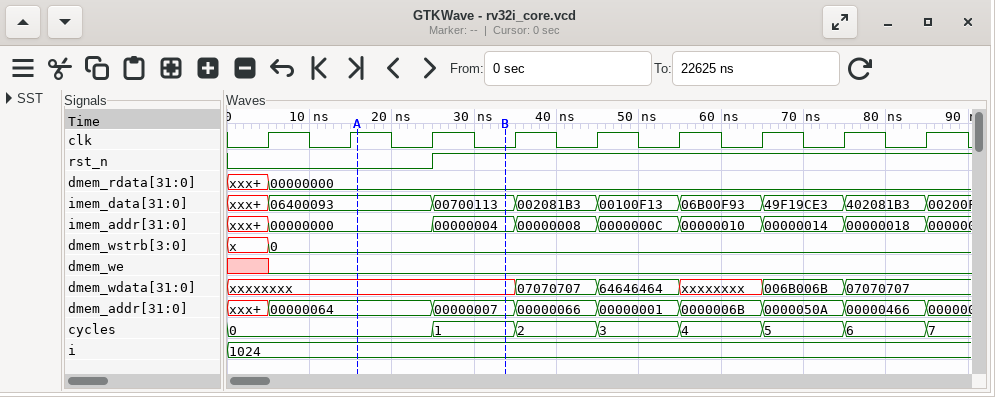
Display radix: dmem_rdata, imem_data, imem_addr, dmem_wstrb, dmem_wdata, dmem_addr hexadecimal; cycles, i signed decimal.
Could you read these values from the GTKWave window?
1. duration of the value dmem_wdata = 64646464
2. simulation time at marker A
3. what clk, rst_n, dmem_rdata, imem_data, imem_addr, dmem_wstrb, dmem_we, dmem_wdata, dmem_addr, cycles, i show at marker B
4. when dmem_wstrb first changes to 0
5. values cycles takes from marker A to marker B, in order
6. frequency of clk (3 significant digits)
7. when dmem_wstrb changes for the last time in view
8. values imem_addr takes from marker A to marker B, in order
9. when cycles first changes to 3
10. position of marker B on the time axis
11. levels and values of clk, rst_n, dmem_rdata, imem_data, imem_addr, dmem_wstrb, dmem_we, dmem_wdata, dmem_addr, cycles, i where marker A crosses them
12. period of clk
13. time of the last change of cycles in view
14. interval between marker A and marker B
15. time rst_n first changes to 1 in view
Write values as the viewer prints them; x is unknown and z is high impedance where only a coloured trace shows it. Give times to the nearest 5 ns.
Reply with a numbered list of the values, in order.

1. 10 ns
2. 15 ns
3. clk=0, rst_n=1, dmem_rdata=00000000, imem_data=00700113, imem_addr=00000004, dmem_wstrb=0, dmem_we=0, dmem_wdata=xxxxxxxx, dmem_addr=00000007, cycles=1, i=1024
4. 5 ns
5. 0, 1
6. 100 MHz
7. 5 ns
8. 00000000, 00000004
9. 45 ns
10. 35 ns
11. clk=1, rst_n=0, dmem_rdata=00000000, imem_data=06400093, imem_addr=00000000, dmem_wstrb=0, dmem_we=0, dmem_wdata=xxxxxxxx, dmem_addr=00000064, cycles=0, i=1024
12. 10 ns
13. 85 ns
14. 20 ns
15. 25 ns
